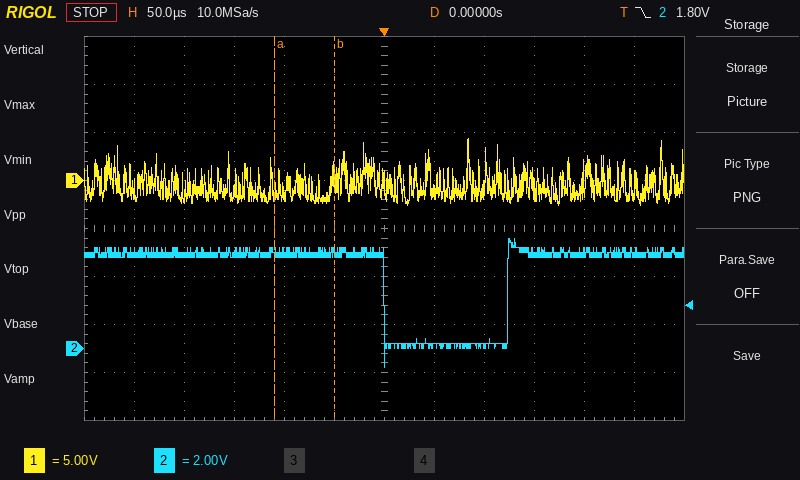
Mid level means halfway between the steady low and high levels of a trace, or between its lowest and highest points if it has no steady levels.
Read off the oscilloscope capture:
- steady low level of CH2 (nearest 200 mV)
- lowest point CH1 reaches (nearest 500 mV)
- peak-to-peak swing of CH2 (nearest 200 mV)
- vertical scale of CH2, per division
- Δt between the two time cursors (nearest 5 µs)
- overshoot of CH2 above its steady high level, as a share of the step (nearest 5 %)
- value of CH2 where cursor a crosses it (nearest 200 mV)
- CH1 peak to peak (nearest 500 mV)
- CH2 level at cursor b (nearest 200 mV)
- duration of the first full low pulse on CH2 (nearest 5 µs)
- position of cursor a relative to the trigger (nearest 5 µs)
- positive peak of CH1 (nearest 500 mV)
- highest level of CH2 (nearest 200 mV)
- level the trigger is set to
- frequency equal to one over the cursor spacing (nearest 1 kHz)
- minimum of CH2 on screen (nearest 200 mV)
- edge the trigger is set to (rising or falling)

200 mV
-2.5 V
5.4 V
2 V
60 µs
20 %
4.0 V
7.0 V
4.0 V
125 µs
-110 µs
4.5 V
4.6 V
1.80 V
17 kHz
-800 mV
falling
